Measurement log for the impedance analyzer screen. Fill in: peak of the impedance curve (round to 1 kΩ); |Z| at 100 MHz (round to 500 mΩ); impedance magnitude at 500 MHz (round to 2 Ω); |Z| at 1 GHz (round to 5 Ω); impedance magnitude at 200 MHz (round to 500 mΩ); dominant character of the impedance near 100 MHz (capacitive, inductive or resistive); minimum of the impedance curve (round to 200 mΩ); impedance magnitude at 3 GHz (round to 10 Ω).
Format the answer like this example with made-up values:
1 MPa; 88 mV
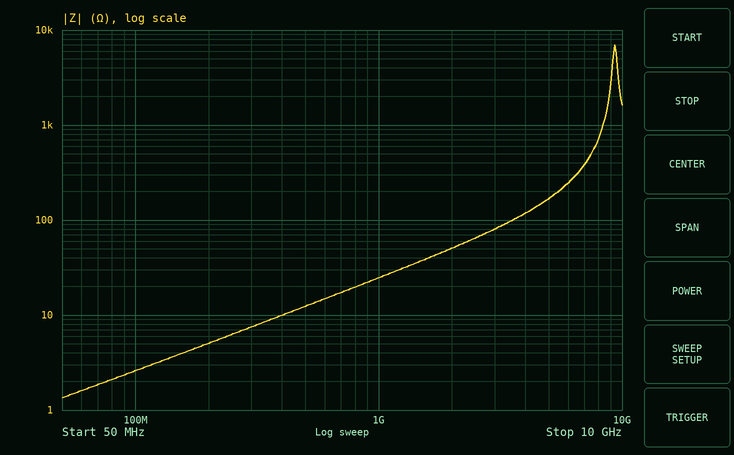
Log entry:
7 kΩ; 2.5 Ω; 12 Ω; 25 Ω; 5.0 Ω; inductive; 1.4 Ω; 80 Ω
